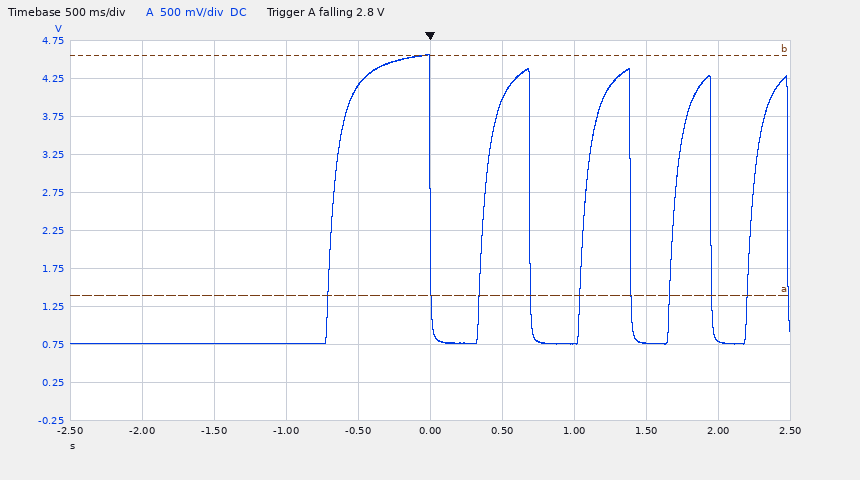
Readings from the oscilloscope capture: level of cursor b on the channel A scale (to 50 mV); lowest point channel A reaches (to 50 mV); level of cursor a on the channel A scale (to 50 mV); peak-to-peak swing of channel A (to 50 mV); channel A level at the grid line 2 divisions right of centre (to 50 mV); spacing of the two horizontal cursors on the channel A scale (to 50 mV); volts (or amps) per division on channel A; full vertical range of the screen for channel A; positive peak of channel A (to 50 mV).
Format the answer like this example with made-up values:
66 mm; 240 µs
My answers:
4.55 V; 750 mV; 1.40 V; 3.80 V; 750 mV; 3.15 V; 500 mV; 5 V; 4.55 V
